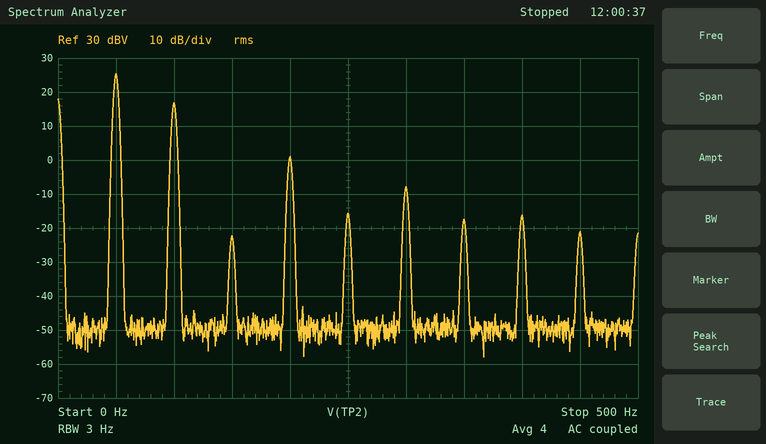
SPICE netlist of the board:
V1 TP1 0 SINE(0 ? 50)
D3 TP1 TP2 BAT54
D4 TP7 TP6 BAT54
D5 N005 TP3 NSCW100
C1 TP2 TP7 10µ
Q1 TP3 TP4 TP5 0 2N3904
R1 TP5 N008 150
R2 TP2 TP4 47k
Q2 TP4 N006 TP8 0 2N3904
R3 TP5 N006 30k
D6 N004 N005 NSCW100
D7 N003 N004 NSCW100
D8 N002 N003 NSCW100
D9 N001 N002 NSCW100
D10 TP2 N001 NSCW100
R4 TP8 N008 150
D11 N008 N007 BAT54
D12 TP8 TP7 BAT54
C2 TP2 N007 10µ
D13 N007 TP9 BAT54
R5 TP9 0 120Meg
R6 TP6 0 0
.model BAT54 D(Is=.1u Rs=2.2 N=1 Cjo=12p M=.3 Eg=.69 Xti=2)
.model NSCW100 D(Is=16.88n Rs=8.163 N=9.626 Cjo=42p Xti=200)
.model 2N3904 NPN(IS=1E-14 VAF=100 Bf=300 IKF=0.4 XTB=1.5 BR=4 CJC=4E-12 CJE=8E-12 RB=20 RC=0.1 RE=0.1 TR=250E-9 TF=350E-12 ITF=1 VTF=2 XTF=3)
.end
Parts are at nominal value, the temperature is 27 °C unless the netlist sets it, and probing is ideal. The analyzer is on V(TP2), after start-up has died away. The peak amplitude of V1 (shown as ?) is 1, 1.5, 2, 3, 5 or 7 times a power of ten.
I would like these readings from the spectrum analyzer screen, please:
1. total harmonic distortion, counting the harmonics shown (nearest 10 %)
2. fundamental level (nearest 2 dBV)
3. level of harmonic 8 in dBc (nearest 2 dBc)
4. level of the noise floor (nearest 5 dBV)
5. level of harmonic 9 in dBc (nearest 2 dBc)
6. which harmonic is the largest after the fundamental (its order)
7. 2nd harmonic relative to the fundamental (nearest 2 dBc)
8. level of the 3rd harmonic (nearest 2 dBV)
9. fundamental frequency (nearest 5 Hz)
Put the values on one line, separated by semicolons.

40 %; 26 dBV; -42 dBc; -50 dBV; -46 dBc; 2; -8 dBc; -22 dBV; 50 Hz
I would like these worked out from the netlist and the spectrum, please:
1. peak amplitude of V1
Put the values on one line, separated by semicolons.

50 V
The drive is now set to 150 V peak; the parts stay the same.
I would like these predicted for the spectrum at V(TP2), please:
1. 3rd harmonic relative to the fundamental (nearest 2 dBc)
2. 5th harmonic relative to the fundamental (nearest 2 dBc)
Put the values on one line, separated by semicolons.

-36 dBc; -46 dBc
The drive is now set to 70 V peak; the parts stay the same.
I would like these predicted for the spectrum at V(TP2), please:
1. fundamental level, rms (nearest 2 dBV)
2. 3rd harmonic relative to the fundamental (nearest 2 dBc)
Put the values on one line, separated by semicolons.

28 dBV; -46 dBc
